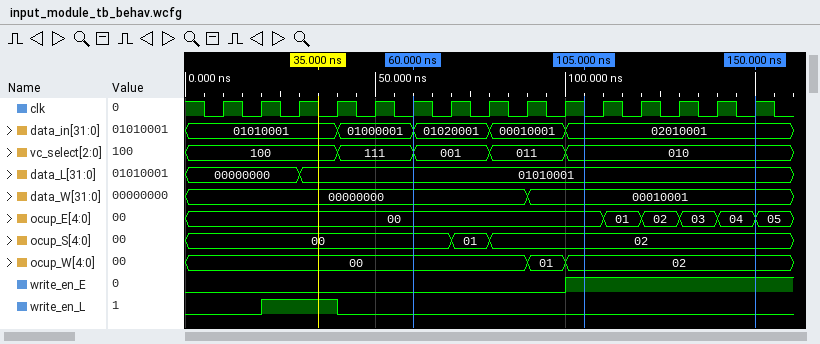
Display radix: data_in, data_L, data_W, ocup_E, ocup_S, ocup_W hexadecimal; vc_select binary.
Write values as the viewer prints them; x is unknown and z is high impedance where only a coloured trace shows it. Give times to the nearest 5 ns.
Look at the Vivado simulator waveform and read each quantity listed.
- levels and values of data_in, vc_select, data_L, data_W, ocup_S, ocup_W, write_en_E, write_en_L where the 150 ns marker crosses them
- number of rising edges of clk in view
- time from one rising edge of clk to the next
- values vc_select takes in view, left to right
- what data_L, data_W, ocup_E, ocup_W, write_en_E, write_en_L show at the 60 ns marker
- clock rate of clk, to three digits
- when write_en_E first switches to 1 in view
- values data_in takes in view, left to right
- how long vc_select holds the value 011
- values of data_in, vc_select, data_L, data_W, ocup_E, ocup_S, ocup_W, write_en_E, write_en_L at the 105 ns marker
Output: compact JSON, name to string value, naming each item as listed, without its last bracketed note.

{"levels and values of data_in, vc_select, data_L, data_W, ocup_S, ocup_W, write_en_E, write_en_L where the 150 ns marker crosses them": "data_in=02010001, vc_select=010, data_L=01010001, data_W=00010001, ocup_S=02, ocup_W=02, write_en_E=1, write_en_L=0", "number of rising edges of clk in view": "15", "time from one rising edge of clk to the next": "10 ns", "values vc_select takes in view, left to right": "100, 111, 001, 011, 010", "what data_L, data_W, ocup_E, ocup_W, write_en_E, write_en_L show at the 60 ns marker": "data_L=01010001, data_W=00000000, ocup_E=00, ocup_W=00, write_en_E=0, write_en_L=0", "clock rate of clk, to three digits": "100 MHz", "when write_en_E first switches to 1 in view": "100 ns", "values data_in takes in view, left to right": "01010001, 01000001, 01020001, 00010001, 02010001", "how long vc_select holds the value 011": "20 ns", "values of data_in, vc_select, data_L, data_W, ocup_E, ocup_S, ocup_W, write_en_E, write_en_L at the 105 ns marker": "data_in=02010001, vc_select=010, data_L=01010001, data_W=00010001, ocup_E=00, ocup_S=02, ocup_W=02, write_en_E=1, write_en_L=0"}
